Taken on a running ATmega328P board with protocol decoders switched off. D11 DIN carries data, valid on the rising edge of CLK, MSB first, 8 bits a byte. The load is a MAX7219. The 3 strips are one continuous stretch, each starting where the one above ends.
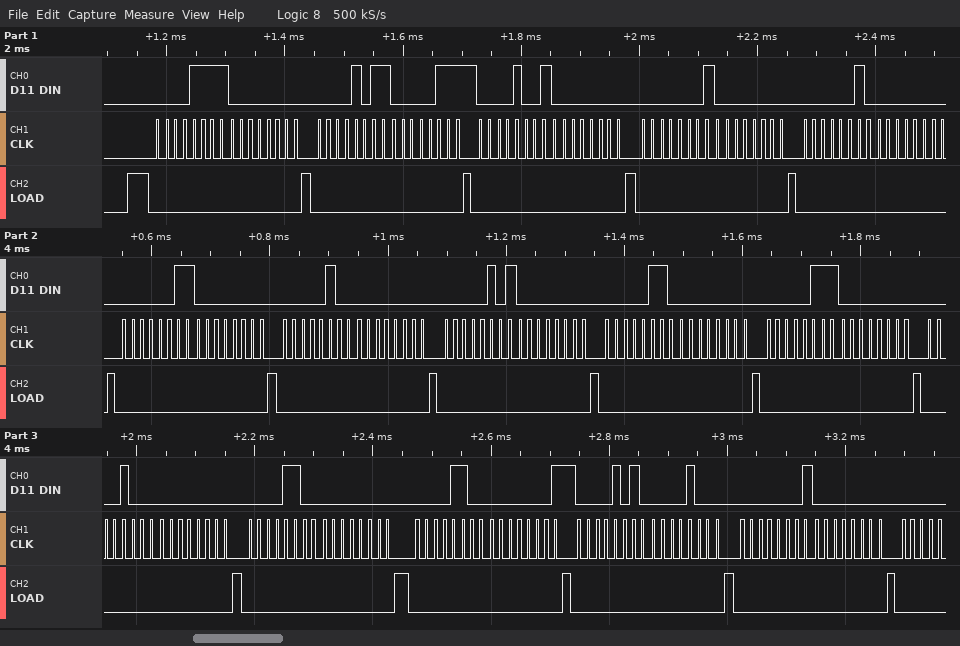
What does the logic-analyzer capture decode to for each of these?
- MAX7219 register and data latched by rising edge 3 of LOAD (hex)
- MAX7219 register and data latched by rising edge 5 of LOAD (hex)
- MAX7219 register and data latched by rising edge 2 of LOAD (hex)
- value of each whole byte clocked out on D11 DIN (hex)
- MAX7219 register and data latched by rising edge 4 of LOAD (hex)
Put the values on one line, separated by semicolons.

register 0xB, data 0x07; register 0x1, data 0x00; register 0xF, data 0x00; 0x0F 0x00 0x0B 0x07 0x09 0x00 0x01 0x00 0x02 0x00 0x03 0x00 0x04 0x00 0x05 0x00 0x06 0x00 0x07 0x00 0x08 0x00 0x0C 0x00 0x0C 0x01 0x0A 0x08 0x01 0x00; register 0x9, data 0x00
